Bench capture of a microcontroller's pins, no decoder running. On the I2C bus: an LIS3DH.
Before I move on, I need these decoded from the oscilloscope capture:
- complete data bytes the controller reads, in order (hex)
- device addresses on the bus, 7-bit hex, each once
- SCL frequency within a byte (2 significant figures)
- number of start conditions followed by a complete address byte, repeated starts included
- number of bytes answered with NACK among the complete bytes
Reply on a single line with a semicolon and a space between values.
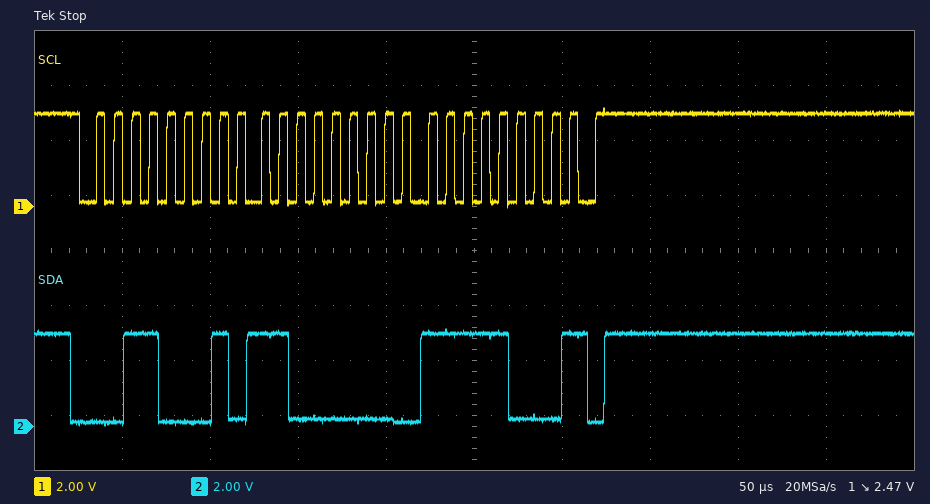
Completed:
C0 F8; 0x18; 100 kHz; 1; 1
